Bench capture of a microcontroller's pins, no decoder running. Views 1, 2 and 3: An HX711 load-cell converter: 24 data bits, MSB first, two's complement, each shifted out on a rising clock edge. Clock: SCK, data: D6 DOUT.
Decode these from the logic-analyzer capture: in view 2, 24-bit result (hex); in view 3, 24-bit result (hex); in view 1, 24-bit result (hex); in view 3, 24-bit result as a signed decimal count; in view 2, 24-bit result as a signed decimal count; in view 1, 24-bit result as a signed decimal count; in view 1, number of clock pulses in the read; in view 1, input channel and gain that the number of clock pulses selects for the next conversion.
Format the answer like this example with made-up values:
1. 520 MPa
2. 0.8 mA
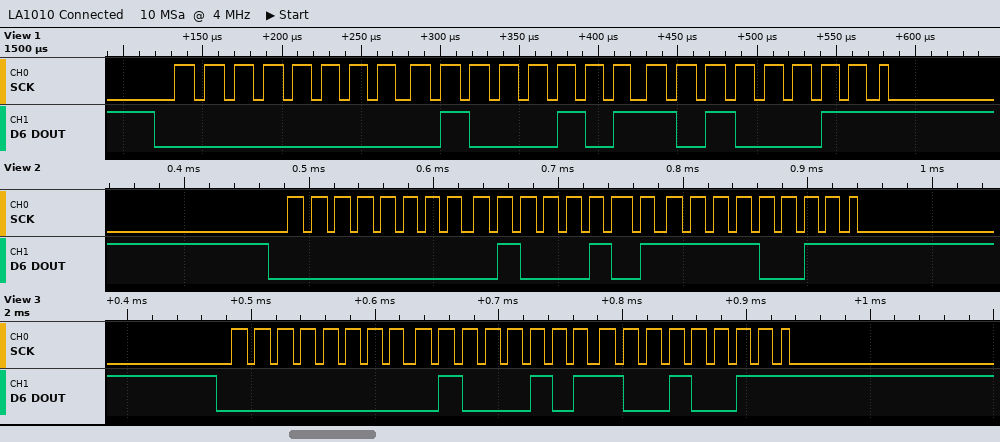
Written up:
1. 0x0045F3
2. 0x004593
3. 0x0045A3
4. 17811
5. 17907
6. 17827
7. 25
8. channel A, gain 128
